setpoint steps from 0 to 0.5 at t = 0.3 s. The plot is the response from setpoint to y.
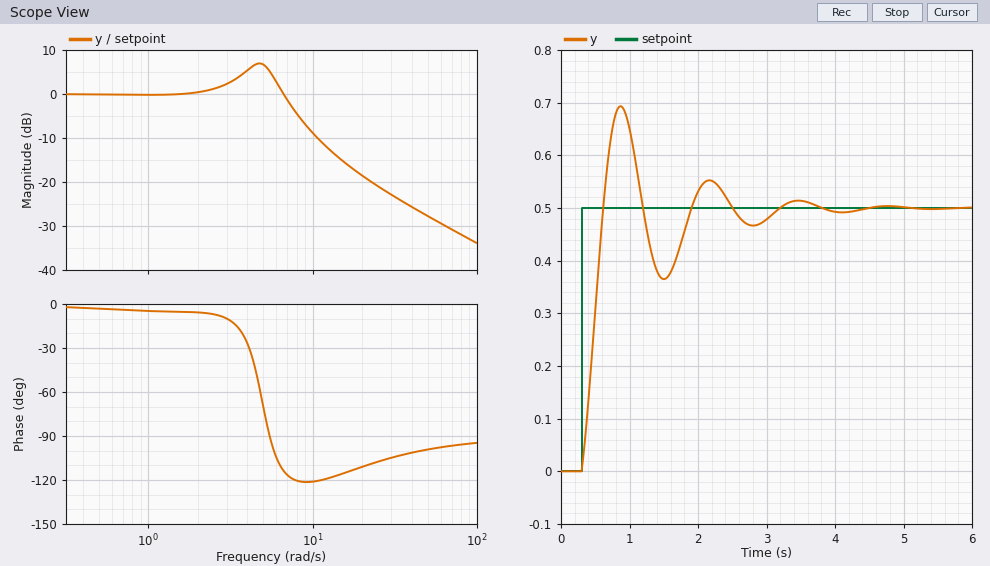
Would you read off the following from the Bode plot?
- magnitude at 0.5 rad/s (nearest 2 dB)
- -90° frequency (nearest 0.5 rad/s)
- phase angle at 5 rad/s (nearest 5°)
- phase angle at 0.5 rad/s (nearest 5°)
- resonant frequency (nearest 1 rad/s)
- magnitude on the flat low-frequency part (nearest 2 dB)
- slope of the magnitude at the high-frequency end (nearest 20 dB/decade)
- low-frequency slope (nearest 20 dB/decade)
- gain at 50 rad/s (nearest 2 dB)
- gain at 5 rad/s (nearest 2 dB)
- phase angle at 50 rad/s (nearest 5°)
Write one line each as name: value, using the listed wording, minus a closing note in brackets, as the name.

magnitude at 0.5 rad/s: 0 dB
-90° frequency: 5.5 rad/s
phase angle at 5 rad/s: -70°
phase angle at 0.5 rad/s: -5°
resonant frequency: 5 rad/s
magnitude on the flat low-frequency part: 0 dB
slope of the magnitude at the high-frequency end: -20 dB/decade
low-frequency slope: 0 dB/decade
gain at 50 rad/s: -28 dB
gain at 5 rad/s: 6 dB
phase angle at 50 rad/s: -100°
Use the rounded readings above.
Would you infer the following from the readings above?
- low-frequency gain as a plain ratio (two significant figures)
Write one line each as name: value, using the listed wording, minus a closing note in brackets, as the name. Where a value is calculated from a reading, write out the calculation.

low-frequency gain as a plain ratio: 10^(0 / 20) = 1.0
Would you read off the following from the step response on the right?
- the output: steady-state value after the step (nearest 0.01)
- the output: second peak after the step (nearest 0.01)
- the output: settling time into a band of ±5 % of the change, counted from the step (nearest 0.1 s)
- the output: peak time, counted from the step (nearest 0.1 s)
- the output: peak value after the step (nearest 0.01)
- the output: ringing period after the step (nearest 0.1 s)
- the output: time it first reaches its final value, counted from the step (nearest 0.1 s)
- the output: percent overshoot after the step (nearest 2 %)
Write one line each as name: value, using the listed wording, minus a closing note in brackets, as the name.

the output: steady-state value after the step: 0.50
the output: second peak after the step: 0.55
the output: settling time into a band of ±5 % of the change, counted from the step: 2.7 s
the output: peak time, counted from the step: 0.6 s
the output: peak value after the step: 0.69
the output: ringing period after the step: 1.3 s
the output: time it first reaches its final value, counted from the step: 0.3 s
the output: percent overshoot after the step: 38 %
